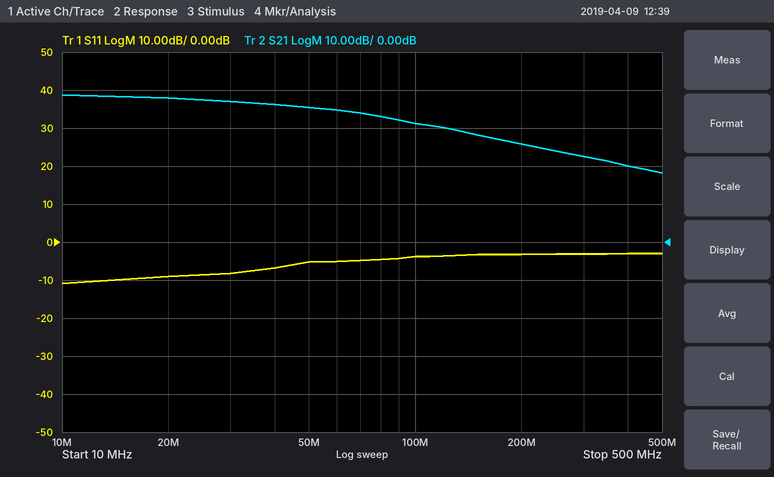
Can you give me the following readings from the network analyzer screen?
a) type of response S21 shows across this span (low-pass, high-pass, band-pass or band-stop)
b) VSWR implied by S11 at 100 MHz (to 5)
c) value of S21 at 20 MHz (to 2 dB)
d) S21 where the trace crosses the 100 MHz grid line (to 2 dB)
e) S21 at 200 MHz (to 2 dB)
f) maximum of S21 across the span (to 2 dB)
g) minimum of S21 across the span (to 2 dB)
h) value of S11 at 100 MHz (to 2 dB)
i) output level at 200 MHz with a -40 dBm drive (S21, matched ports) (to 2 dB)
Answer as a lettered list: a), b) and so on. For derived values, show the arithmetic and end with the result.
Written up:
a) low-pass
b) |Γ| = 10^(-4/20) = 0.6310; VSWR = (1 + 0.6310)/(1 − 0.6310) ≈ 4.42, so 5 to the nearest 5
c) 38 dB
d) 32 dB
e) 26 dB
f) 38 dB
g) 18 dB
h) -4 dB
i) -40 dBm + (26 dB) = -14 dBm
